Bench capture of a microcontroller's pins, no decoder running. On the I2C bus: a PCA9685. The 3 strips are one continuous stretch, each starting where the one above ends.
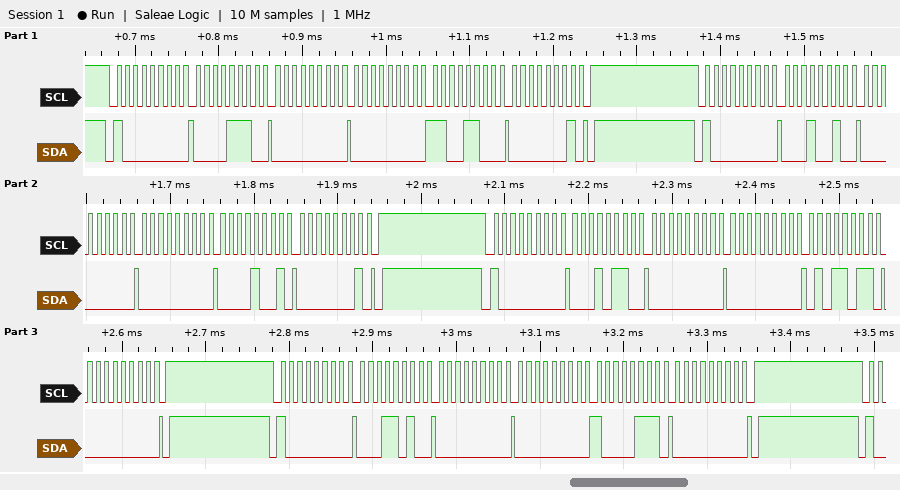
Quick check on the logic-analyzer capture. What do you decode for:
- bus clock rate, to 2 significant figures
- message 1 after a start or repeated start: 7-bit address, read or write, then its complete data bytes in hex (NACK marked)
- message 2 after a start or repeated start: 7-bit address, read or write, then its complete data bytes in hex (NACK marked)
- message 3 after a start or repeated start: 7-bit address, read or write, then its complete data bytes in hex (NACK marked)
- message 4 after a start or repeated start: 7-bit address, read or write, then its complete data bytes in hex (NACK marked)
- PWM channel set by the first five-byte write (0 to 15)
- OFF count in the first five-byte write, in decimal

100 kHz
0x40 write: 0E 00 00 CC 01
0x40 write: 12 00 00 09 01
0x40 write: 16 00 00 5B 00
0x40 write: 1A 00 00 87 00
2
460
